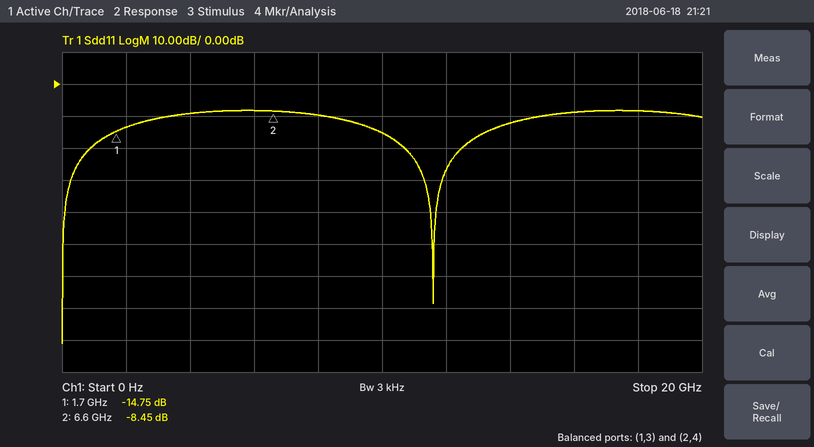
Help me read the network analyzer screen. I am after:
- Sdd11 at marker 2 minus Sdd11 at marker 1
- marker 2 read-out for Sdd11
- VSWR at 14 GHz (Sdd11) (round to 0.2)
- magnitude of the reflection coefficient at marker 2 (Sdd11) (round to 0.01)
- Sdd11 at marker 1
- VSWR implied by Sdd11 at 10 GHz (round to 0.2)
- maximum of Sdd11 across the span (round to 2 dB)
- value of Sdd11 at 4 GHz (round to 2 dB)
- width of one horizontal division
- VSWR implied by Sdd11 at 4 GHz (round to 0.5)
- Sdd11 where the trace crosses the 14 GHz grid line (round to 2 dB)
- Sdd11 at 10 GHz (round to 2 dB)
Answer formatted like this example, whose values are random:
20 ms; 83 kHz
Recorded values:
6.30 dB; -8.45 dB; 1.6; 0.38; -14.75 dB; 1.4; -8 dB; -10 dB; 2 GHz; 2.0; -12 dB; -16 dB
